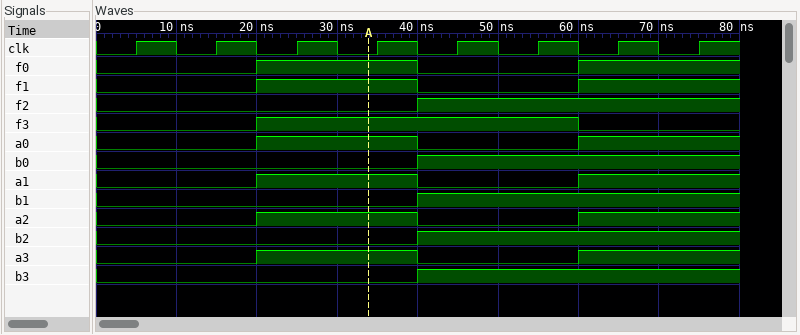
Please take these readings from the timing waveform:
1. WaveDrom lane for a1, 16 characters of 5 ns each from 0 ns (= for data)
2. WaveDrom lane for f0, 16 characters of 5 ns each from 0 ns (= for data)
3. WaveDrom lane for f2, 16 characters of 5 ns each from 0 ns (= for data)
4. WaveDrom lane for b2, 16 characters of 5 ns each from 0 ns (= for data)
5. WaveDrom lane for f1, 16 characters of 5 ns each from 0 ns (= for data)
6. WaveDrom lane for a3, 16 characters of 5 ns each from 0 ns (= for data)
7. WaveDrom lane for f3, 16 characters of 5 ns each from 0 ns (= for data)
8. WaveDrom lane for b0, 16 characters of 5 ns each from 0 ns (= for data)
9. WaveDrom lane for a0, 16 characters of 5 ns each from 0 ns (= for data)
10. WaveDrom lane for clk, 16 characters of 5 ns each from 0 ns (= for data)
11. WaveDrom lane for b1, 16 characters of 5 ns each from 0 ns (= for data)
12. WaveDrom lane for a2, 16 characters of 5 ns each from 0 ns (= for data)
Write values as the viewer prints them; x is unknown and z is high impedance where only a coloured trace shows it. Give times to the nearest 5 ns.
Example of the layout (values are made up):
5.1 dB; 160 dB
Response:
{name: 'a1', wave: '0...1...0...1...'}; {name: 'f0', wave: '0...1...0...1...'}; {name: 'f2', wave: '0.......1.......'}; {name: 'b2', wave: '0.......1.......'}; {name: 'f1', wave: '0...1...0...1...'}; {name: 'a3', wave: '0...1...0...1...'}; {name: 'f3', wave: '0...1.......0...'}; {name: 'b0', wave: '0.......1.......'}; {name: 'a0', wave: '0...1...0...1...'}; {name: 'clk', wave: '0101010101010101'}; {name: 'b1', wave: '0.......1.......'}; {name: 'a2', wave: '0...1...0...1...'}
